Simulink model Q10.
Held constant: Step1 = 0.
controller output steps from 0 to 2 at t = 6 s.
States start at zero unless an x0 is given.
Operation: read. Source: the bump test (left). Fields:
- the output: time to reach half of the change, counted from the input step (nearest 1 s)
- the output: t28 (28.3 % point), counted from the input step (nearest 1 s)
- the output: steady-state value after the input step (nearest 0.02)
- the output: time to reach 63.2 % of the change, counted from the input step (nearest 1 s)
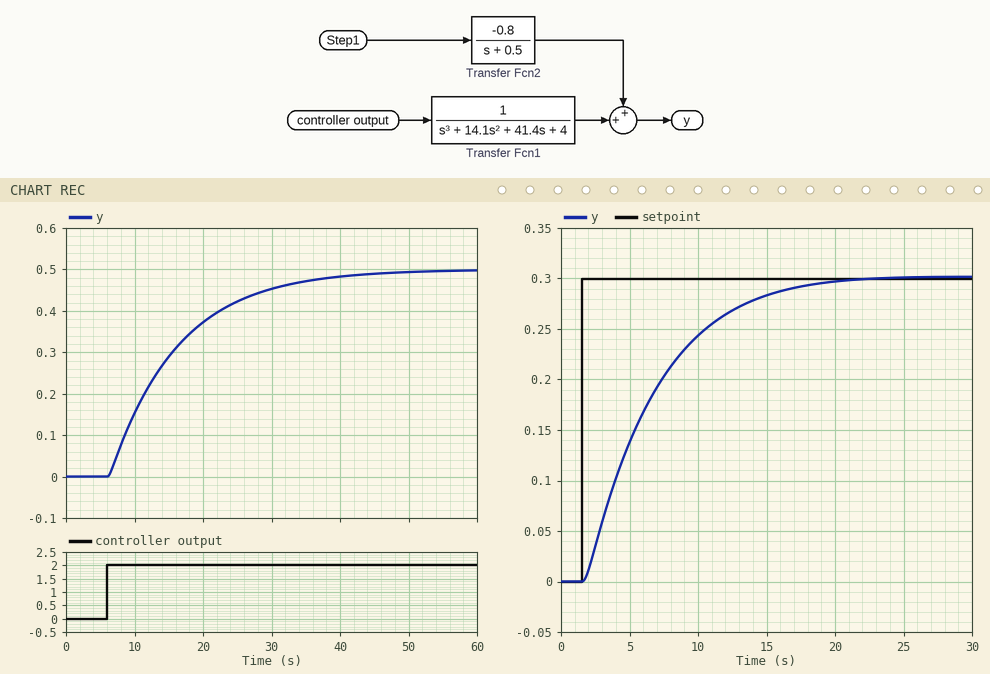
7 s
4 s
0.50
10 s
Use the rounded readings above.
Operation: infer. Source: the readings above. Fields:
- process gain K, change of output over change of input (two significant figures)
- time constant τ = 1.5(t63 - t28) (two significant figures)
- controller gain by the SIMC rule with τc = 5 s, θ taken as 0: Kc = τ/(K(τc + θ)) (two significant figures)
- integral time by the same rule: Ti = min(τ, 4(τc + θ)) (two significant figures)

0.25
9.0 s
7.2
9.0 s
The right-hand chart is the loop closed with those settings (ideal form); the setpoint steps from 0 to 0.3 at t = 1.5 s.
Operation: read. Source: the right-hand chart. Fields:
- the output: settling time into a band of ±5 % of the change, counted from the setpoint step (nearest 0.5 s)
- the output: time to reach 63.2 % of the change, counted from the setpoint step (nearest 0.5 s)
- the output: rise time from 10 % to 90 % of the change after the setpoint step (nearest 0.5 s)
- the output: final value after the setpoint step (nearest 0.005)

14.0 s
5.5 s
10.5 s
0.300
